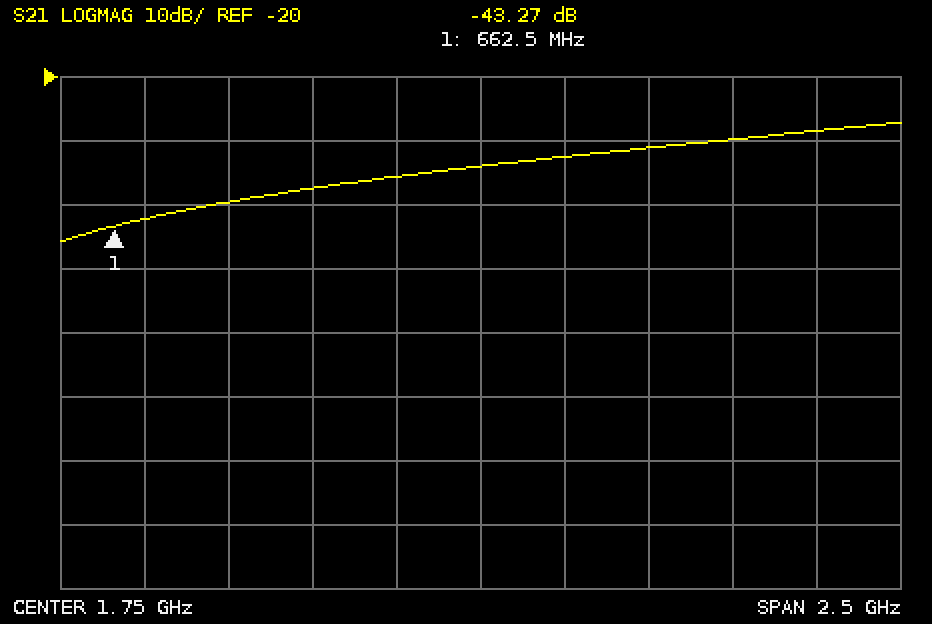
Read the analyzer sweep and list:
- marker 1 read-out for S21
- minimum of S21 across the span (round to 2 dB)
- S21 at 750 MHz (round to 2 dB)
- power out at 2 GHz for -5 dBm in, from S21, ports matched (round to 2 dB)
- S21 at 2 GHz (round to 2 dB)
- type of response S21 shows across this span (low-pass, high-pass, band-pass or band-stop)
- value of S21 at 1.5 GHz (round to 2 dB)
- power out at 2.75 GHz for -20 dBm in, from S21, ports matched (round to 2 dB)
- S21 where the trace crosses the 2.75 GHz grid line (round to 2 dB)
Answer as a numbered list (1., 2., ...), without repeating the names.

1. -43.27 dB
2. -46 dB
3. -42 dB
4. -38 dBm
5. -32 dB
6. high-pass
7. -36 dB
8. -48 dBm
9. -28 dB
